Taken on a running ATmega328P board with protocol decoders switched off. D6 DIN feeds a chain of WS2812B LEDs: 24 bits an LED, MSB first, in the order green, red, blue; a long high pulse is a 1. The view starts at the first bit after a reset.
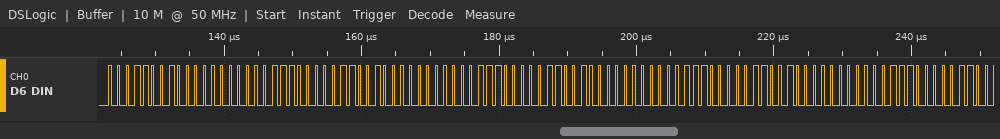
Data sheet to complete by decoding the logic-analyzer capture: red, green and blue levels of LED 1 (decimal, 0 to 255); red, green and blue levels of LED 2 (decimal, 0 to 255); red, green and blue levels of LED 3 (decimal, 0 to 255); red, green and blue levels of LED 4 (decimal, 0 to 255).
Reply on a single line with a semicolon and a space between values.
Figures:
0, 25, 28; 0, 25, 28; 0, 25, 28; 0, 25, 28
